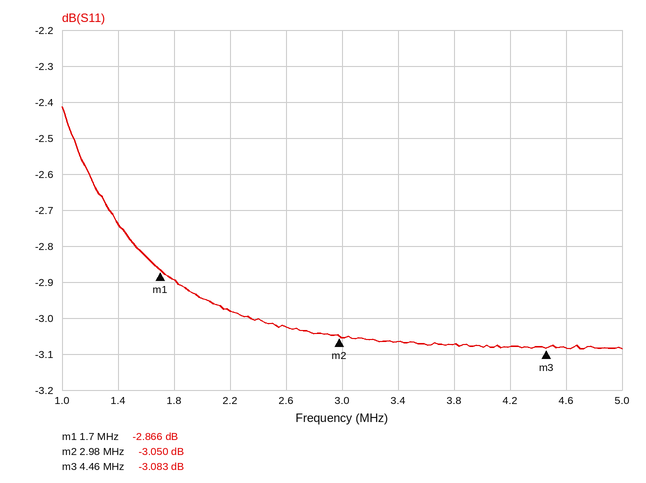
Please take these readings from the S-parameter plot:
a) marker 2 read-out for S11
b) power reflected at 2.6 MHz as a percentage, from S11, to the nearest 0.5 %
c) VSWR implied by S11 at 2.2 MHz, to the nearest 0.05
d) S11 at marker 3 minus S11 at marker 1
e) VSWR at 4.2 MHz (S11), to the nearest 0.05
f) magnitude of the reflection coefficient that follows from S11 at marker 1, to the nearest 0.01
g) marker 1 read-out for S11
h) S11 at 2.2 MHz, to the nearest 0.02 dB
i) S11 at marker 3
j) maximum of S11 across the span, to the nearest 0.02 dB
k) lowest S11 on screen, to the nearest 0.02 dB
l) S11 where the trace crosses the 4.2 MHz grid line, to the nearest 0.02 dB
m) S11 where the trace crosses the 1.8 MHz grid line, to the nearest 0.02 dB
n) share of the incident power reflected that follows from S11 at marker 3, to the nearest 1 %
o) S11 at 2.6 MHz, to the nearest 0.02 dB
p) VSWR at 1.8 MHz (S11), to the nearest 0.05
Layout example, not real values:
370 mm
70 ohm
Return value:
-3.050 dB
50.0 %
5.90
-0.217 dB
5.70
0.72
-2.866 dB
-2.98 dB
-3.083 dB
-2.42 dB
-3.08 dB
-3.08 dB
-2.90 dB
49 %
-3.02 dB
6.05
